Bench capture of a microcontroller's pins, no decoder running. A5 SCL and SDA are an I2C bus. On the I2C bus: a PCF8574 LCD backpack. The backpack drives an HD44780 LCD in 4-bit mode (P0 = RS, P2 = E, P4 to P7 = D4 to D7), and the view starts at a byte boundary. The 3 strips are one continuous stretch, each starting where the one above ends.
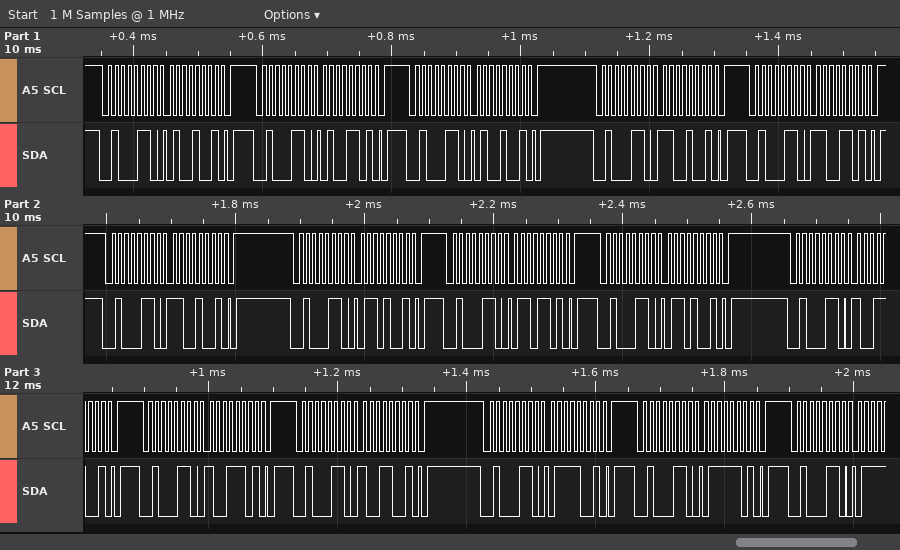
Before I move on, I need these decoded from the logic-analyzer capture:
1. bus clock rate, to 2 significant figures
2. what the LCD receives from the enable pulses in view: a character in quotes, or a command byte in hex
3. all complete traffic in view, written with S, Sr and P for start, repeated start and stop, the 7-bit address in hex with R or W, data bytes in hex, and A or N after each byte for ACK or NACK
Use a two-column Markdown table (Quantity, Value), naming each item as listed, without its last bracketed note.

| Quantity | Value |
|---|---|
| bus clock rate, to 2 significant figures | 100 kHz |
| what the LCD receives from the enable pulses in view: a character in quotes, or a command byte in hex | 'L' 'i' |
| all complete traffic in view, written with S, Sr and P for start, repeated start and stop, the 7-bit address in hex with R or W, data bytes in hex, and A or N after each byte for ACK or NACK | S 23W A 49 A P S 23W A 4D A P S 23W A 49 A P S 23W A C9 A P S 23W A CD A P S 23W A C9 A P S 23W A 69 A P S 23W A 6D A P S 23W A 69 A P S 23W A 99 A P S 23W A 9D A P S 23W A 99 A P S 23W A 79 A P S 23W A 7D A P S 23W A |
